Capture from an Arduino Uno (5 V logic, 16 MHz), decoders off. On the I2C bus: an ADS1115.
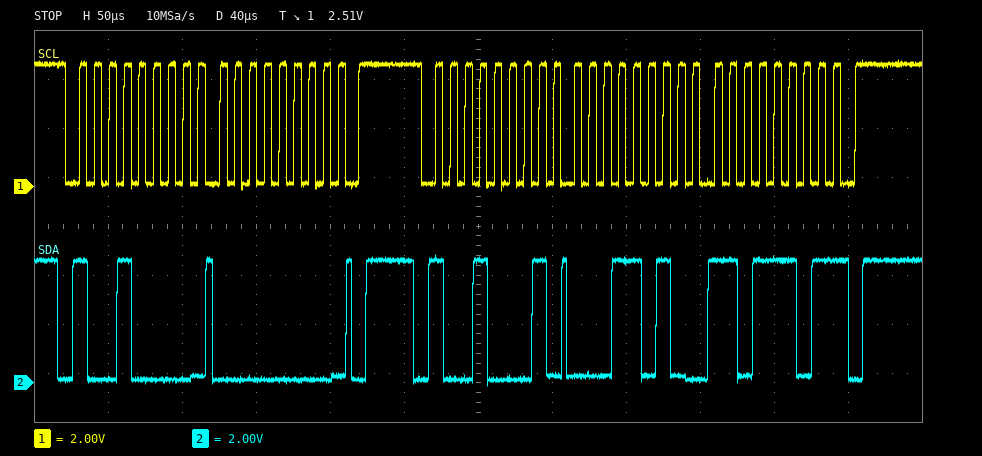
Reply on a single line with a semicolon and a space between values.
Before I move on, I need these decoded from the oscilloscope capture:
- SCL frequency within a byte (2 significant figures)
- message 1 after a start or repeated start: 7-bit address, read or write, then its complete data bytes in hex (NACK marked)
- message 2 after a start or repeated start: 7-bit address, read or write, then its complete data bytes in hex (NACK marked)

100 kHz; 0x48 write: 00; 0x48 read: 1A DD NACK
